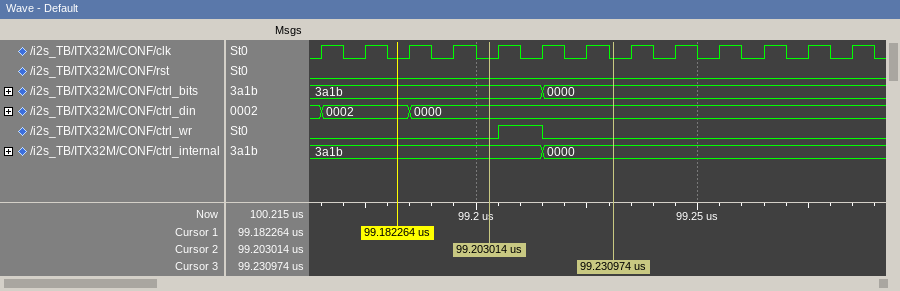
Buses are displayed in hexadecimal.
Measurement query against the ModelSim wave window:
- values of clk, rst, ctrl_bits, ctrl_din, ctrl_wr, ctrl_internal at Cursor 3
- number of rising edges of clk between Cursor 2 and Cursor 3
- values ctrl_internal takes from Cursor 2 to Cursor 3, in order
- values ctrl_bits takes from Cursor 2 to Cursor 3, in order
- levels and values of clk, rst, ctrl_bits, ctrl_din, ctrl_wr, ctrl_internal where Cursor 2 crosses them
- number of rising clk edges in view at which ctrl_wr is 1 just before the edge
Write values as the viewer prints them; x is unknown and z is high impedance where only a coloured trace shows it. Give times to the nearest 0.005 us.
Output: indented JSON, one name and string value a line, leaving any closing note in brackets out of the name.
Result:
{
  "values of clk, rst, ctrl_bits, ctrl_din, ctrl_wr, ctrl_internal at Cursor 3": "clk=0, rst=0, ctrl_bits=0000, ctrl_din=0000, ctrl_wr=0, ctrl_internal=0000",
  "number of rising edges of clk between Cursor 2 and Cursor 3": "3",
  "values ctrl_internal takes from Cursor 2 to Cursor 3, in order": "3a1b, 0000",
  "values ctrl_bits takes from Cursor 2 to Cursor 3, in order": "3a1b, 0000",
  "levels and values of clk, rst, ctrl_bits, ctrl_din, ctrl_wr, ctrl_internal where Cursor 2 crosses them": "clk=0, rst=0, ctrl_bits=3a1b, ctrl_din=0000, ctrl_wr=0, ctrl_internal=3a1b",
  "number of rising clk edges in view at which ctrl_wr is 1 just before the edge": "1"
}
